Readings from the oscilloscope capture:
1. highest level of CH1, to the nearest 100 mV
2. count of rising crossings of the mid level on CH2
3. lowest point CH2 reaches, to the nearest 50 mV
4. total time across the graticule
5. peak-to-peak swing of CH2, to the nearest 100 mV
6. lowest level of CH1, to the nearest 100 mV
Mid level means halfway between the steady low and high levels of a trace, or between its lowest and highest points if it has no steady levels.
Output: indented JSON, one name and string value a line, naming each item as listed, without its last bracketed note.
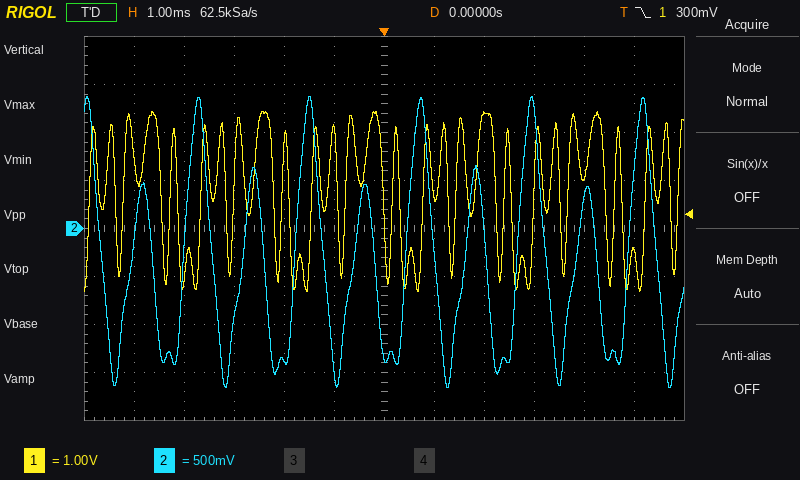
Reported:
{
  "highest level of CH1, to the nearest 100 mV": "2.4 V",
  "count of rising crossings of the mid level on CH2": "10",
  "lowest point CH2 reaches, to the nearest 50 mV": "-1.65 V",
  "total time across the graticule": "12 ms",
  "peak-to-peak swing of CH2, to the nearest 100 mV": "3.00 V",
  "lowest level of CH1, to the nearest 100 mV": "-1.3 V"
}
